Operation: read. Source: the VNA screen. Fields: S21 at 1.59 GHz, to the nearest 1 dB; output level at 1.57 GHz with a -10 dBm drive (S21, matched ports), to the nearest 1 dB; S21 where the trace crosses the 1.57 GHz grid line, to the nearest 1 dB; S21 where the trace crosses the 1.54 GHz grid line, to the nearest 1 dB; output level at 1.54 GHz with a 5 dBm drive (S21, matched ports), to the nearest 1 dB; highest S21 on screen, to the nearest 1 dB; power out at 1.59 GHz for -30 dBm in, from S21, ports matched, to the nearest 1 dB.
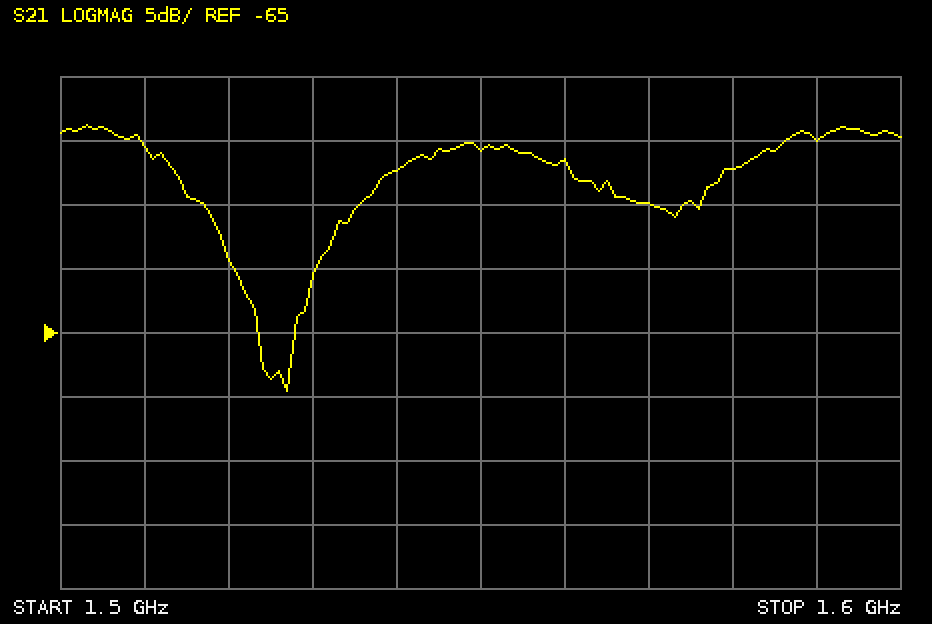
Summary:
-50 dB
-65 dBm
-55 dB
-52 dB
-47 dBm
-49 dB
-80 dBm
